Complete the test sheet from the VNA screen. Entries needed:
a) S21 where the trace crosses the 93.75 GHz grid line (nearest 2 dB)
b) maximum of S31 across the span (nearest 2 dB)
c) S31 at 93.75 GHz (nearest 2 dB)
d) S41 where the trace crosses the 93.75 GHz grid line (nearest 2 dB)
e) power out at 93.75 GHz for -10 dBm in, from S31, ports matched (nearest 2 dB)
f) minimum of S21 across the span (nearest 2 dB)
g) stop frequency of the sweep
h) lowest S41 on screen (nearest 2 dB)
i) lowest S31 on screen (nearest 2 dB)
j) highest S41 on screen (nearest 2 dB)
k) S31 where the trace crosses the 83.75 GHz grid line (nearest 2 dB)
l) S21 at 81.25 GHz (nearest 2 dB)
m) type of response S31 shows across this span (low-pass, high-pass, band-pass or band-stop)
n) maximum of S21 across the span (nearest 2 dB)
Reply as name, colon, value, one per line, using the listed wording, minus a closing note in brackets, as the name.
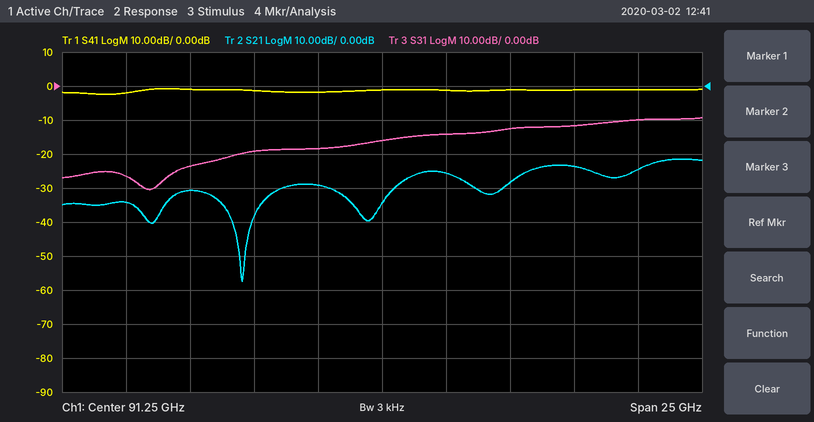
S21 where the trace crosses the 93.75 GHz grid line: -26 dB
maximum of S31 across the span: -10 dB
S31 at 93.75 GHz: -14 dB
S41 where the trace crosses the 93.75 GHz grid line: -2 dB
power out at 93.75 GHz for -10 dBm in, from S31, ports matched: -24 dBm
minimum of S21 across the span: -58 dB
stop frequency of the sweep: 103.75 GHz
lowest S41 on screen: -2 dB
lowest S31 on screen: -30 dB
highest S41 on screen: 0 dB
S31 where the trace crosses the 83.75 GHz grid line: -24 dB
S21 at 81.25 GHz: -34 dB
type of response S31 shows across this span: high-pass
maximum of S21 across the span: -22 dB
